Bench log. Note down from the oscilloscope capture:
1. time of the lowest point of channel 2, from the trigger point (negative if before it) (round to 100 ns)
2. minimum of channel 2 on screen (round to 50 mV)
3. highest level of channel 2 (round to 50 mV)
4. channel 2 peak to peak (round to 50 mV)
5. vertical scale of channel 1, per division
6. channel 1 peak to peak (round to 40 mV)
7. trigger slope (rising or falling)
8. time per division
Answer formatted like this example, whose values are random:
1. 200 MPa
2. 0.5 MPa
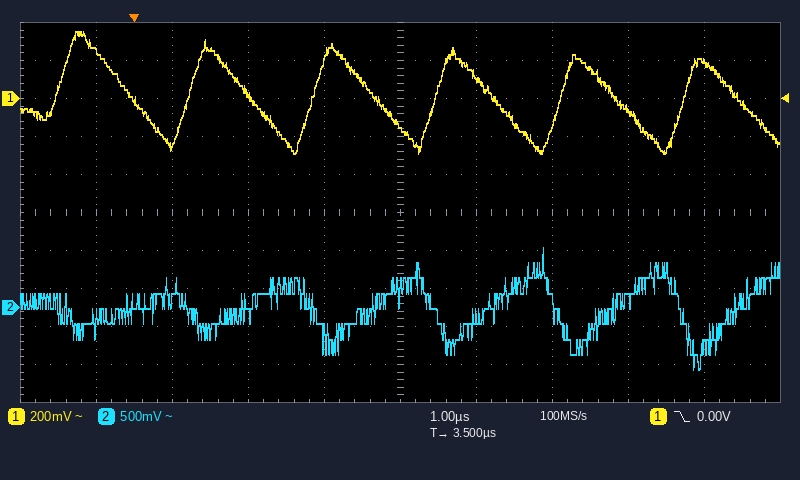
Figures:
1. +7.4 µs
2. -800 mV
3. 800 mV
4. 1.60 V
5. 200 mV
6. 640 mV
7. falling
8. 1 µs
